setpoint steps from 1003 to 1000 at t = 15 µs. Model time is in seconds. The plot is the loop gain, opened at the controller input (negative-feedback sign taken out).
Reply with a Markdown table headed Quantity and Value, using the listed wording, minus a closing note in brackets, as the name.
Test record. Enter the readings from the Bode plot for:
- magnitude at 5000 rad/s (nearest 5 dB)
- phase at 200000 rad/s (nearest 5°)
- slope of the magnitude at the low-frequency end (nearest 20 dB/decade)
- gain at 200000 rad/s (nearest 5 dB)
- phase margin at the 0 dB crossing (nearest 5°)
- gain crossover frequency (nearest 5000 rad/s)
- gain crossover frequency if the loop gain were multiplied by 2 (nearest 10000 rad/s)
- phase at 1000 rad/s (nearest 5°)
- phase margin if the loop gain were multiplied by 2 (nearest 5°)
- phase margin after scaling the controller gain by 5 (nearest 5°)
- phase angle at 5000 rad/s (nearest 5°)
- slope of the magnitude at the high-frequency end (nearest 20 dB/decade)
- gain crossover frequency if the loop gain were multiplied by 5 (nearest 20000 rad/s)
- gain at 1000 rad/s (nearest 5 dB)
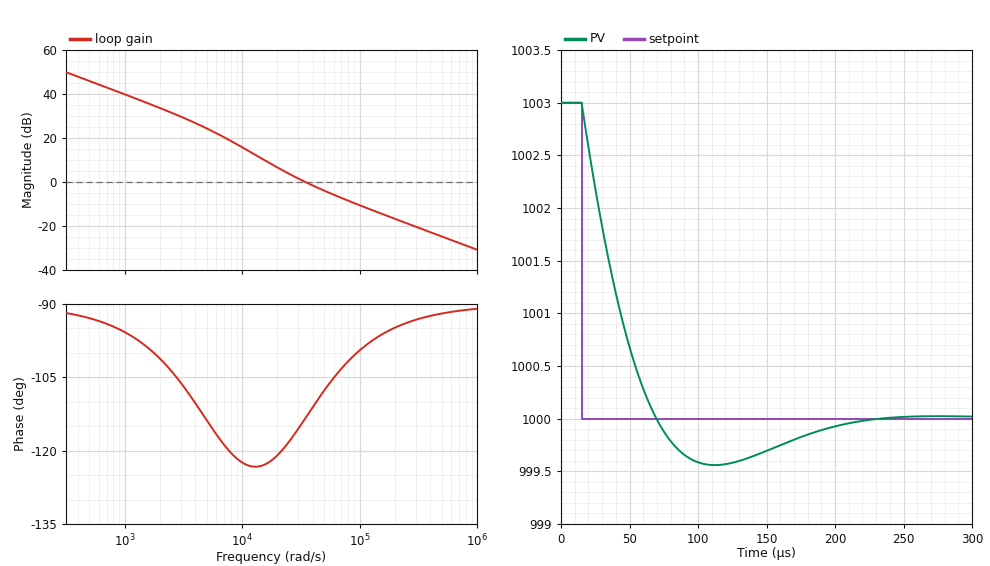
| Quantity | Value |
|---|---|
| magnitude at 5000 rad/s | 25 dB |
| phase at 200000 rad/s | -95° |
| slope of the magnitude at the low-frequency end | -20 dB/decade |
| gain at 200000 rad/s | -15 dB |
| phase margin at the 0 dB crossing | 65° |
| gain crossover frequency | 35000 rad/s |
| gain crossover frequency if the loop gain were multiplied by 2 | 60000 rad/s |
| phase at 1000 rad/s | -95° |
| phase margin if the loop gain were multiplied by 2 | 75° |
| phase margin after scaling the controller gain by 5 | 85° |
| phase angle at 5000 rad/s | -115° |
| slope of the magnitude at the high-frequency end | -20 dB/decade |
| gain crossover frequency if the loop gain were multiplied by 5 | 140000 rad/s |
| gain at 1000 rad/s | 40 dB |
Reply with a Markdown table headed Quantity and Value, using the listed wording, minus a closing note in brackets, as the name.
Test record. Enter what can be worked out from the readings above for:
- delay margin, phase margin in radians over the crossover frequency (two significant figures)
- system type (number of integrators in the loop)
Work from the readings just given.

| Quantity | Value |
|---|---|
| delay margin, phase margin in radians over the crossover frequency | 0.000032 s |
| system type | 1 |
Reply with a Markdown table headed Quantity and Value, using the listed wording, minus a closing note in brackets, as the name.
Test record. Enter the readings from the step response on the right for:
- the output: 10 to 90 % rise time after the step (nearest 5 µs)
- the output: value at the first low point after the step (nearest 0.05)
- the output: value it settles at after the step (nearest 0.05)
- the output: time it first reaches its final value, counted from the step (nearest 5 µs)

| Quantity | Value |
|---|---|
| the output: 10 to 90 % rise time after the step | 40 µs |
| the output: value at the first low point after the step | 999.55 |
| the output: value it settles at after the step | 1000.00 |
| the output: time it first reaches its final value, counted from the step | 55 µs |
